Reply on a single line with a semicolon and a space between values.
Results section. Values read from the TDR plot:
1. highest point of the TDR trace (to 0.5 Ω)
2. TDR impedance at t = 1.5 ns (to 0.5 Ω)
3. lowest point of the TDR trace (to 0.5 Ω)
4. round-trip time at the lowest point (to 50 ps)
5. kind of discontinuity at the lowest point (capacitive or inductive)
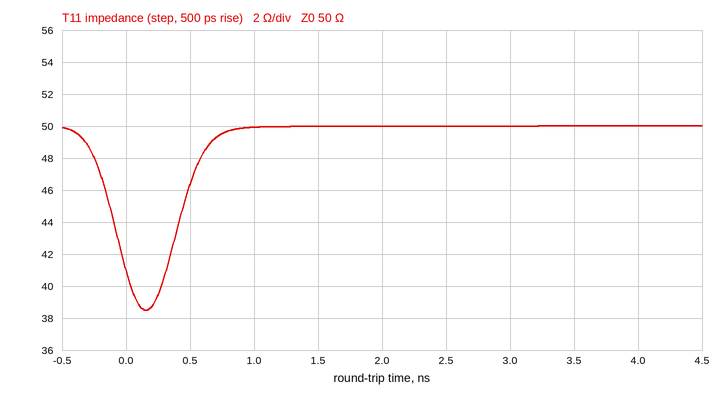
50.0 Ω; 50.0 Ω; 38.5 Ω; 150 ps; capacitive
